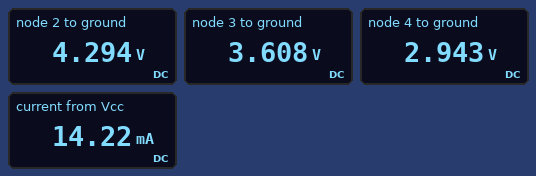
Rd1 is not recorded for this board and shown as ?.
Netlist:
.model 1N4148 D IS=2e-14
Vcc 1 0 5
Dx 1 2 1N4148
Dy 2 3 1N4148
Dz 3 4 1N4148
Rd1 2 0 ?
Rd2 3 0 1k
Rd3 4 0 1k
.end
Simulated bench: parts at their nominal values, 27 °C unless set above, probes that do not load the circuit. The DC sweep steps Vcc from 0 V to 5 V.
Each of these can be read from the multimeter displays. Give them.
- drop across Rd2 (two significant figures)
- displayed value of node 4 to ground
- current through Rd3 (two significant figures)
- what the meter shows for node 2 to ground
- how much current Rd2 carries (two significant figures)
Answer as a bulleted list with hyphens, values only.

- 3.6 V
- 2.943 V
- 2.9 mA
- 4.294 V
- 3.6 mA
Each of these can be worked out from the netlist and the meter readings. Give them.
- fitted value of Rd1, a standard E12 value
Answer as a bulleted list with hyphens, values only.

- 560 Ω
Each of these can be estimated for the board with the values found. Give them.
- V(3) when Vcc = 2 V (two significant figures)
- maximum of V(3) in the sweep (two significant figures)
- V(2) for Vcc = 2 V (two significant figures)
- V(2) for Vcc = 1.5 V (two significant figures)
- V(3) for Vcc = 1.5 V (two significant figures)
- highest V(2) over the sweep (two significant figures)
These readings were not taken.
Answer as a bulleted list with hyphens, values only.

- 700 mV
- 3.6 V
- 1.3 V
- 850 mV
- 250 mV
- 4.3 V
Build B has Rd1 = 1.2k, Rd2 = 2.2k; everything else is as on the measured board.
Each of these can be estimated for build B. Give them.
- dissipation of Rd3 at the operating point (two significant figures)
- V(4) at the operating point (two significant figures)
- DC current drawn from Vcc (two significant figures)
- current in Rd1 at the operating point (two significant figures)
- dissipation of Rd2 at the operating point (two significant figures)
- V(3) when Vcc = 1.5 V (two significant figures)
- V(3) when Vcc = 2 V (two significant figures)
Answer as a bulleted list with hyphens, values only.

- 8.8 mW
- 3.0 V
- 8.2 mA
- 3.6 mA
- 6.0 mW
- 280 mV
- 730 mV
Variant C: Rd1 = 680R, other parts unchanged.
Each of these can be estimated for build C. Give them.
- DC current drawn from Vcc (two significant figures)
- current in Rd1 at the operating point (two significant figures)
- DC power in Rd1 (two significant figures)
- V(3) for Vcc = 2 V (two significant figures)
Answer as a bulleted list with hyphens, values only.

- 13 mA
- 6.3 mA
- 27 mW
- 700 mV
